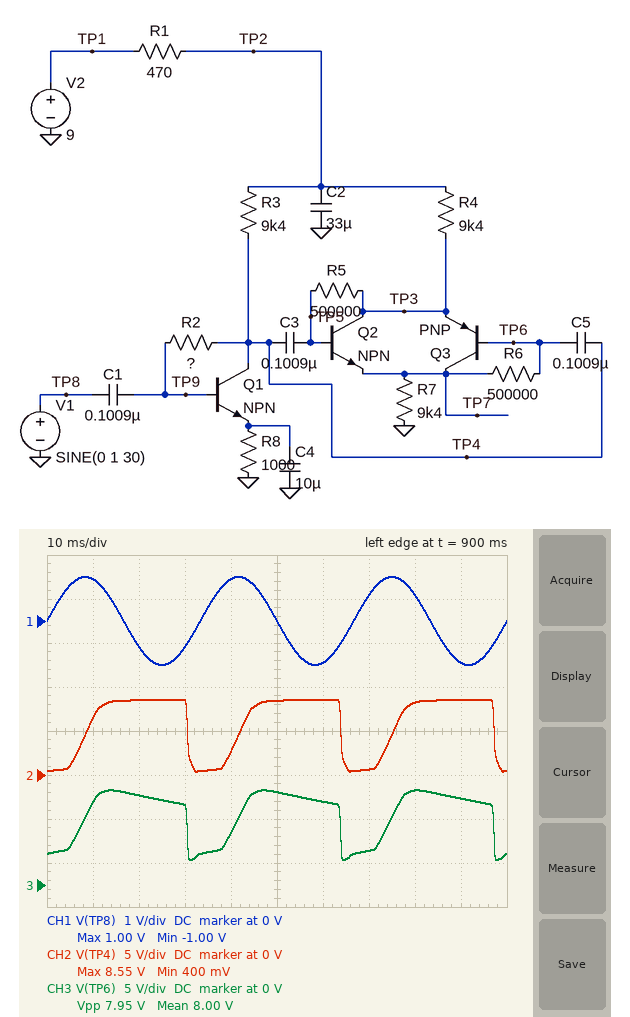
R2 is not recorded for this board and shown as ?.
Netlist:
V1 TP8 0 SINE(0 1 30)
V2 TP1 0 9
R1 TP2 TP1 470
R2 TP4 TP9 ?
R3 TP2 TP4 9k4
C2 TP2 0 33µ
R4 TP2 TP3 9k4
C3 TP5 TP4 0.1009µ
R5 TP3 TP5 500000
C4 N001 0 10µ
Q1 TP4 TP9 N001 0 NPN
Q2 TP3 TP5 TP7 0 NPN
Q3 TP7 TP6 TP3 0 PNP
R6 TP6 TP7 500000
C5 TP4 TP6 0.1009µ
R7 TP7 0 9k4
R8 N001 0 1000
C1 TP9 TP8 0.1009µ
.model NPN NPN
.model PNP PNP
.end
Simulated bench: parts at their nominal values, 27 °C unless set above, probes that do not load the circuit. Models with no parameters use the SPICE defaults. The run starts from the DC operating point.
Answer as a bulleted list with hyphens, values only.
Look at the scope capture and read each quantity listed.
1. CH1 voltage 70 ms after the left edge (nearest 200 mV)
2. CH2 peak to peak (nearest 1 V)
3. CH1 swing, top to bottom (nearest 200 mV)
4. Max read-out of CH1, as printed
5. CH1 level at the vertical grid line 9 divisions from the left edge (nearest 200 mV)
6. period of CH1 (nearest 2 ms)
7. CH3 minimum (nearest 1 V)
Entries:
- 600 mV
- 8 V
- 2.0 V
- 1.00 V
- -1.0 V
- 34 ms
- 3 V
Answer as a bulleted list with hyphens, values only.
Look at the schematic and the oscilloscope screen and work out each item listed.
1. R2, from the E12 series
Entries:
- 1.5 MΩ
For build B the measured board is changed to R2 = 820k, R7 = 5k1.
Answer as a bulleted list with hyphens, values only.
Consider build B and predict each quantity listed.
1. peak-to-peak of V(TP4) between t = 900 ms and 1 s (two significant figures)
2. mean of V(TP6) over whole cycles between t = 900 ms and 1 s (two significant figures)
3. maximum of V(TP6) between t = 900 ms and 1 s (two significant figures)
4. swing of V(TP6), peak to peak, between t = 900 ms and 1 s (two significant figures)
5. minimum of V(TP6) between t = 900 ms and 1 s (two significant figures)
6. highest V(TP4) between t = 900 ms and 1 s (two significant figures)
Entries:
- 7.9 V
- 6.1 V
- 9.5 V
- 7.5 V
- 2.0 V
- 8.4 V
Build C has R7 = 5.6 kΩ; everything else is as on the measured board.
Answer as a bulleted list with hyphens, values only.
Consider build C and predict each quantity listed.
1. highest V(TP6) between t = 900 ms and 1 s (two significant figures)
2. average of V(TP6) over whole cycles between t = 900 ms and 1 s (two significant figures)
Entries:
- 9.8 V
- 7.0 V
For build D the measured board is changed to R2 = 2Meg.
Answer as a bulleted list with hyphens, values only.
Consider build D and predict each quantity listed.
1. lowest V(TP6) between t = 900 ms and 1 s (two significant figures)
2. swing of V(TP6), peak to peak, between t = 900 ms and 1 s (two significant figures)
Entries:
- 2.6 V
- 8.2 V
